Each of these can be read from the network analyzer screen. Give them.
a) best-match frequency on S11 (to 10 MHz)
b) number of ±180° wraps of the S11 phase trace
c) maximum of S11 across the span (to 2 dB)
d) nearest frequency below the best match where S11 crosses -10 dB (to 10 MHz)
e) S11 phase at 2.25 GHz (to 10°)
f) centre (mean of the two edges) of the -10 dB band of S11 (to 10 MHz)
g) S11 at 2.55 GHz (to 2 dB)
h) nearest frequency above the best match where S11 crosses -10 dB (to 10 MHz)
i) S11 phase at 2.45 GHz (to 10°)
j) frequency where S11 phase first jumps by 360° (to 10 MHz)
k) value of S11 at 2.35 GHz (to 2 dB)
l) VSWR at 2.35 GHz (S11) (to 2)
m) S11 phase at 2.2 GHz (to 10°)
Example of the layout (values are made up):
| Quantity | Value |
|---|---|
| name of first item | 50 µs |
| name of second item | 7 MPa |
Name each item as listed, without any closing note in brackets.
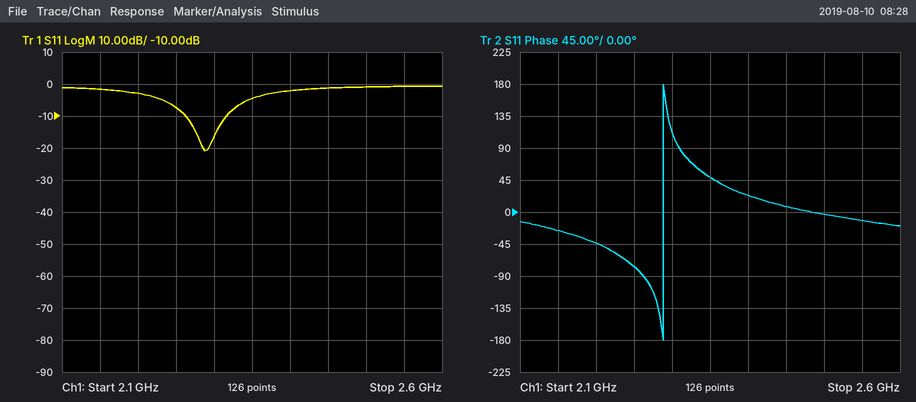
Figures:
| Quantity | Value |
|---|---|
| best-match frequency on S11 | 2.29 GHz |
| number of ±180° wraps of the S11 phase trace | 1 |
| maximum of S11 across the span | 0 dB |
| nearest frequency below the best match where S11 crosses -10 dB | 2.26 GHz |
| S11 phase at 2.25 GHz | -80° |
| centre (mean of the two edges) of the -10 dB band of S11 | 2.29 GHz |
| S11 at 2.55 GHz | 0 dB |
| nearest frequency above the best match where S11 crosses -10 dB | 2.32 GHz |
| S11 phase at 2.45 GHz | 10° |
| frequency where S11 phase first jumps by 360° | 2.29 GHz |
| value of S11 at 2.35 GHz | -4 dB |
| VSWR at 2.35 GHz (S11) | 4 |
| S11 phase at 2.2 GHz | -40° |
